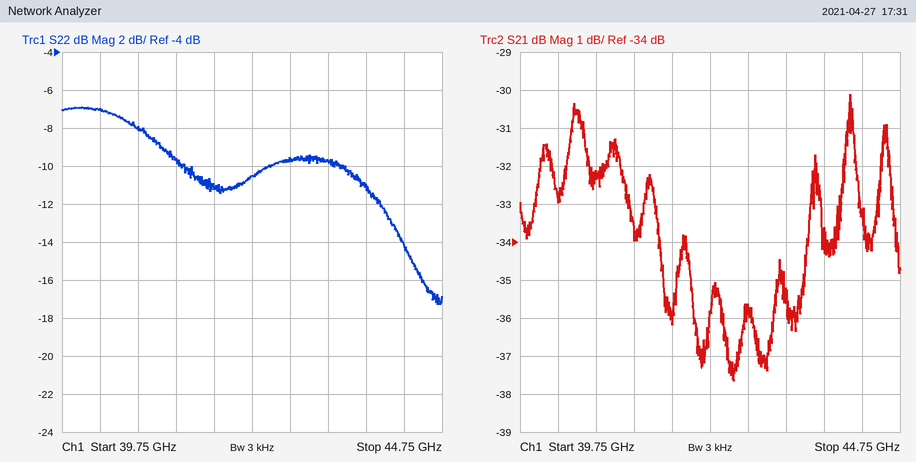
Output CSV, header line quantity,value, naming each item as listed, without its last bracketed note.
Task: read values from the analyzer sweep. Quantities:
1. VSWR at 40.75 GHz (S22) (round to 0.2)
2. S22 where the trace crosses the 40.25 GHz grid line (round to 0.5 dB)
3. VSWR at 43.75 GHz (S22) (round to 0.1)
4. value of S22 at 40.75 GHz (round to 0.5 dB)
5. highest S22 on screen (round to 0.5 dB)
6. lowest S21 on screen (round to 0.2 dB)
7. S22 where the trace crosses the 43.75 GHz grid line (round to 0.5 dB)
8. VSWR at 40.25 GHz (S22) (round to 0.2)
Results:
quantity,value
VSWR at 40.75 GHz (S22),2.4
S22 where the trace crosses the 40.25 GHz grid line,-7.0 dB
VSWR at 43.75 GHz (S22),1.8
value of S22 at 40.75 GHz,-8.0 dB
highest S22 on screen,-7.0 dB
lowest S21 on screen,-37.6 dB
S22 where the trace crosses the 43.75 GHz grid line,-11.0 dB
VSWR at 40.25 GHz (S22),2.6
